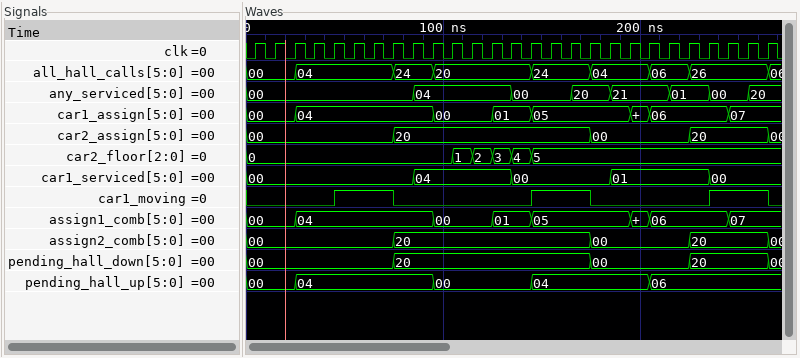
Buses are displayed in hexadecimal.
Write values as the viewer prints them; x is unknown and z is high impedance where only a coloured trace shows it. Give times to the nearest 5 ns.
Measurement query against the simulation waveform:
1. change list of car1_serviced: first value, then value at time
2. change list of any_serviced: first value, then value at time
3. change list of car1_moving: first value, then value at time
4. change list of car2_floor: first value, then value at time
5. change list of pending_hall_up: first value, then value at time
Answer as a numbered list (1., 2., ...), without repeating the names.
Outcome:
1. 00, 04 at 85 ns, 00 at 135 ns, 01 at 185 ns, 00 at 235 ns
2. 00, 04 at 85 ns, 00 at 135 ns, 20 at 165 ns, 21 at 185 ns, 01 at 215 ns, 00 at 235 ns, 20 at 255 ns
3. 0, 1 at 45 ns, 0 at 75 ns, 1 at 145 ns, 0 at 175 ns, 1 at 235 ns, 0 at 265 ns
4. 0, 1 at 105 ns, 2 at 115 ns, 3 at 125 ns, 4 at 135 ns, 5 at 145 ns
5. 00, 04 at 25 ns, 00 at 95 ns, 04 at 145 ns, 06 at 205 ns
